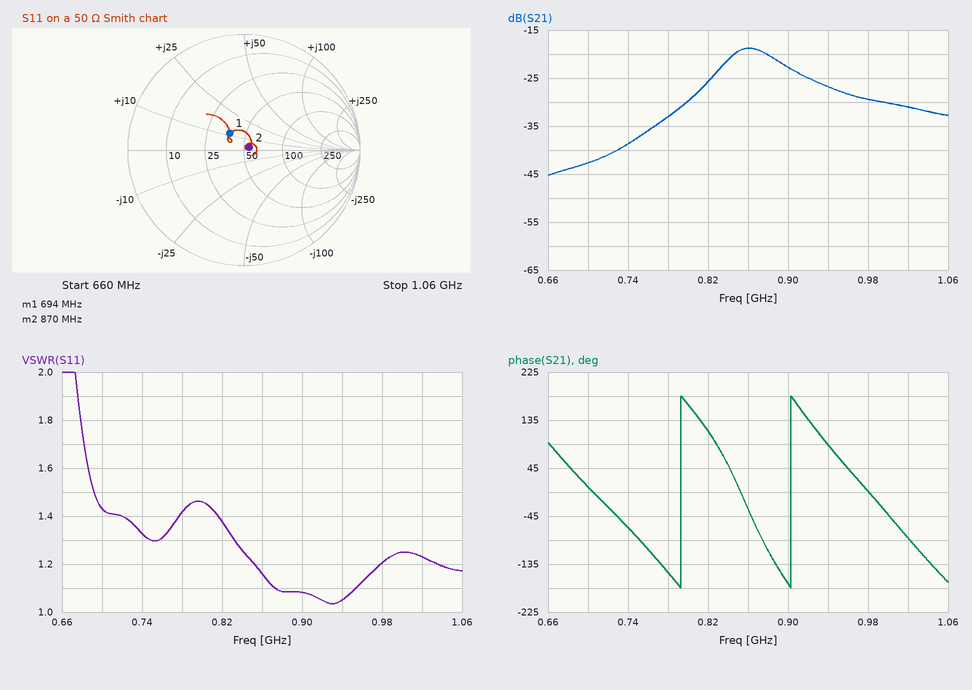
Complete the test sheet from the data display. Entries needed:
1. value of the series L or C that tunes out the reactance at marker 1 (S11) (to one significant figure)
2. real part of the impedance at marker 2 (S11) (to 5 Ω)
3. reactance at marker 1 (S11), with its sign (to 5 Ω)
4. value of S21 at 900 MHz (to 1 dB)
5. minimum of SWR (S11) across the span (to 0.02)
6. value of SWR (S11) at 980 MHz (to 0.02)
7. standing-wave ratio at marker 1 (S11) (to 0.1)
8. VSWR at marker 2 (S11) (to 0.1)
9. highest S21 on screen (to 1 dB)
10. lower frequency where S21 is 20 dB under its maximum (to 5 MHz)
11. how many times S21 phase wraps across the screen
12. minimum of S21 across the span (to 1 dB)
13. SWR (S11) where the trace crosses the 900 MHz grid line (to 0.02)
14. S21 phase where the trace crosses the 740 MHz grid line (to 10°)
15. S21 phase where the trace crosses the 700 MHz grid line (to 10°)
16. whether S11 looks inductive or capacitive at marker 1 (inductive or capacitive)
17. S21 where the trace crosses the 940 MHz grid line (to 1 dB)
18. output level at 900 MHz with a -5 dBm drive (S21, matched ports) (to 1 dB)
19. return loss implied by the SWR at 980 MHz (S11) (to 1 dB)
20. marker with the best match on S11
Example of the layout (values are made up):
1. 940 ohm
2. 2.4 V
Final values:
1. 20 pF
2. 55 Ω
3. +10 Ω
4. -23 dB
5. 1.04
6. 1.20
7. 1.5
8. 1.1
9. -19 dB
10. 740 MHz
11. 2
12. -45 dB
13. 1.08
14. -70°
15. 10°
16. inductive
17. -27 dB
18. -28 dBm
19. 21 dB
20. marker 2
